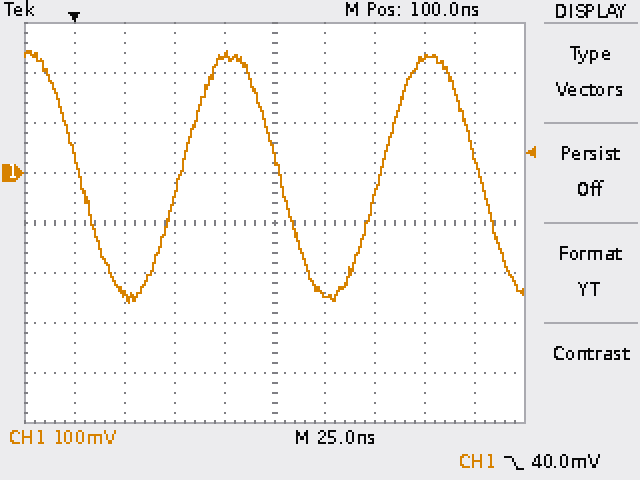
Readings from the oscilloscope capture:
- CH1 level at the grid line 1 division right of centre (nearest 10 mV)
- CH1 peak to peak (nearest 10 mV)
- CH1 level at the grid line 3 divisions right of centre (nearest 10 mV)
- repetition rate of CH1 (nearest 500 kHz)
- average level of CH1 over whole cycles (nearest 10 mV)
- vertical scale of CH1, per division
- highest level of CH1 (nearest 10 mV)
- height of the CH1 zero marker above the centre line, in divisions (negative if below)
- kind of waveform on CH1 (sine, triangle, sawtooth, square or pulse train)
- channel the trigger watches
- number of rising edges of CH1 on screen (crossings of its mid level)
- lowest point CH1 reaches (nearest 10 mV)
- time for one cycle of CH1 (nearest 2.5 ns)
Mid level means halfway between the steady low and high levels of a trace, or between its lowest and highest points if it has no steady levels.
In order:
-240 mV
500 mV
230 mV
10.0 MHz
-10 mV
100 mV
240 mV
+1.0 div
sine
CH1
2
-260 mV
100.0 ns
